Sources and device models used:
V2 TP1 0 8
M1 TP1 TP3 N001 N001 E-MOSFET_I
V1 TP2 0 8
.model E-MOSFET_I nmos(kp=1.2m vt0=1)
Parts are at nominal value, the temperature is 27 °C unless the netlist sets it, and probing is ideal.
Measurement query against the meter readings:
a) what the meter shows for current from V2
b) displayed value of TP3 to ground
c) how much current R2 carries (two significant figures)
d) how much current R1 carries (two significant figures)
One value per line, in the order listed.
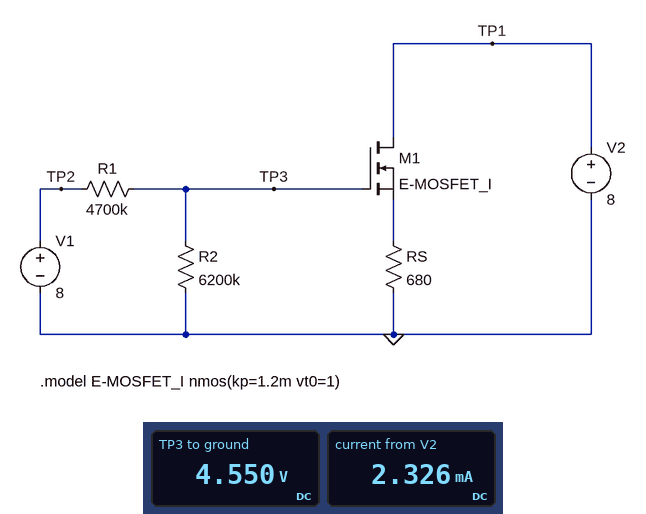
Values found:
2.326 mA
4.550 V
730 nA
730 nA
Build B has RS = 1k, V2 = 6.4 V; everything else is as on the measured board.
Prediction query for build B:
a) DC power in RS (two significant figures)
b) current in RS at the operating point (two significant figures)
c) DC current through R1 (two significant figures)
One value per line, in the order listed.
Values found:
3.3 mW
1.8 mA
730 nA
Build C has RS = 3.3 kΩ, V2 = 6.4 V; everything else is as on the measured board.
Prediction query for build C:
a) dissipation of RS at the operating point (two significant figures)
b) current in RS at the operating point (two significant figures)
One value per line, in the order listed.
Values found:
1.8 mW
740 µA
